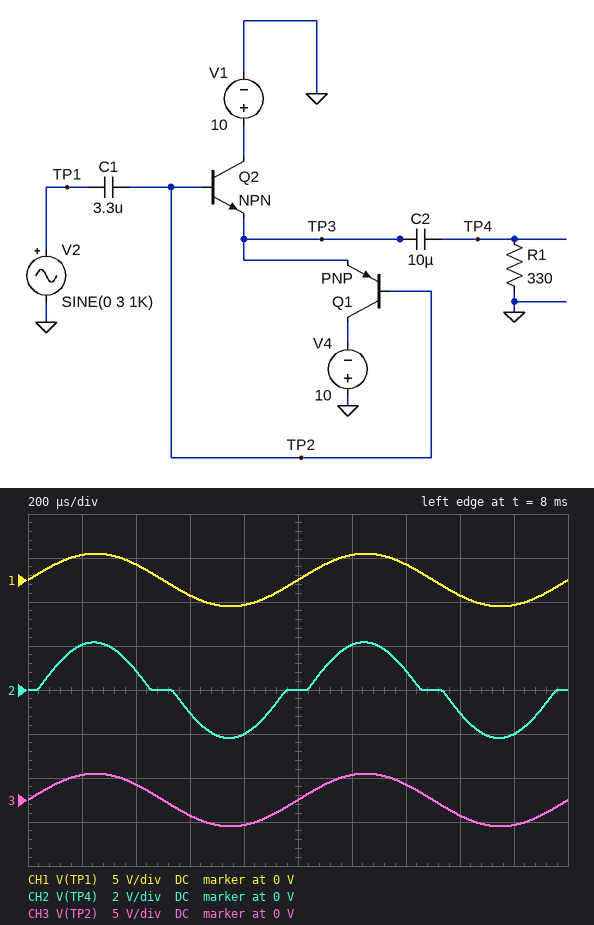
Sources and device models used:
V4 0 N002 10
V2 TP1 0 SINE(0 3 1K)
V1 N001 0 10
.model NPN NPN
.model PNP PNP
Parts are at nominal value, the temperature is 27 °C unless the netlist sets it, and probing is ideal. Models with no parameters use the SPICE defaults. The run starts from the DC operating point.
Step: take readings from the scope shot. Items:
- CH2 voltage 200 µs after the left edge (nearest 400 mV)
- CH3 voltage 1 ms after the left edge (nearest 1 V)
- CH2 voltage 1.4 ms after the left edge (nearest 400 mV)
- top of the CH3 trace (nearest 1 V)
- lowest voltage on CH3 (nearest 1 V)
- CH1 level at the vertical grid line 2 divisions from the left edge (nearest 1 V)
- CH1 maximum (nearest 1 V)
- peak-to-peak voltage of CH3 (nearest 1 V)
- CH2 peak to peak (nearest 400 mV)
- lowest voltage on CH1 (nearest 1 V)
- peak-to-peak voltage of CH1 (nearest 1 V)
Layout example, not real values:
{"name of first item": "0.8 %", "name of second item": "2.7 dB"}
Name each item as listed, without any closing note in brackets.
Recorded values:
{"CH2 voltage 200 µs after the left edge": "2.0 V", "CH3 voltage 1 ms after the left edge": "0 V", "CH2 voltage 1.4 ms after the left edge": "800 mV", "top of the CH3 trace": "3 V", "lowest voltage on CH3": "-3 V", "CH1 level at the vertical grid line 2 divisions from the left edge": "2 V", "CH1 maximum": "3 V", "peak-to-peak voltage of CH3": "6 V", "CH2 peak to peak": "4.4 V", "lowest voltage on CH1": "-3 V", "peak-to-peak voltage of CH1": "6 V"}
